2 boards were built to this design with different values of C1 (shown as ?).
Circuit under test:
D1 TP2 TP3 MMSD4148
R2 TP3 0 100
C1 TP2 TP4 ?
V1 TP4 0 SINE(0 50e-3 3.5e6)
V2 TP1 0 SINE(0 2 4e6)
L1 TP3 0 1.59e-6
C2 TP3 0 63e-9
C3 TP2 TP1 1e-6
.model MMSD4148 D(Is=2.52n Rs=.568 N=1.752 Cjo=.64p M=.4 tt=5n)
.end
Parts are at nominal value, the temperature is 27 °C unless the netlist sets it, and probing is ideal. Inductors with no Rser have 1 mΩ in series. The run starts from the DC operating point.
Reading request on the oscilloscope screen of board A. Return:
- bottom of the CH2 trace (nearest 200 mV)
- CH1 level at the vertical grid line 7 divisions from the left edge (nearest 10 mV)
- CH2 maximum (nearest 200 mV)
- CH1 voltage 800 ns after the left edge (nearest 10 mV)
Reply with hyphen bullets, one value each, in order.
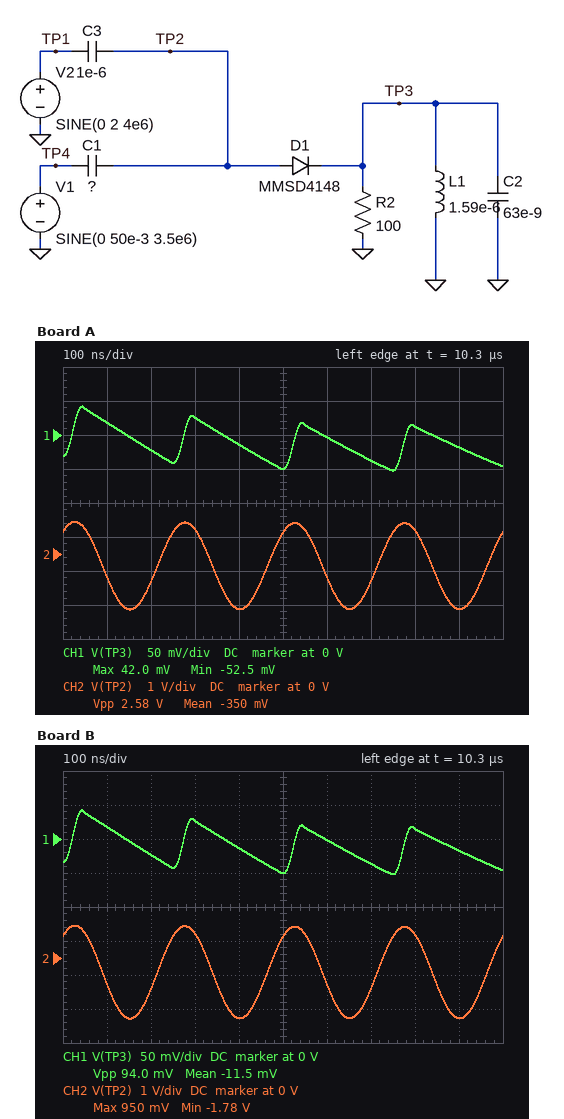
- -1.6 V
- -40 mV
- 1.0 V
- 10 mV
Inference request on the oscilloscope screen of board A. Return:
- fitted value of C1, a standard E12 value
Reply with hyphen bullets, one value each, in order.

- 560 nF
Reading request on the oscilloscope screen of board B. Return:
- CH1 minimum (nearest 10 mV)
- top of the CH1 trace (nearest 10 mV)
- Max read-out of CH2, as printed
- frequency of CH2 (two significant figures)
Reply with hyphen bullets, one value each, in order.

- -50 mV
- 40 mV
- 950 mV
- 4.0 MHz
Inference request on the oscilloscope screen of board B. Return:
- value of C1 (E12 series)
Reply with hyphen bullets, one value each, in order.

- 470 nF
